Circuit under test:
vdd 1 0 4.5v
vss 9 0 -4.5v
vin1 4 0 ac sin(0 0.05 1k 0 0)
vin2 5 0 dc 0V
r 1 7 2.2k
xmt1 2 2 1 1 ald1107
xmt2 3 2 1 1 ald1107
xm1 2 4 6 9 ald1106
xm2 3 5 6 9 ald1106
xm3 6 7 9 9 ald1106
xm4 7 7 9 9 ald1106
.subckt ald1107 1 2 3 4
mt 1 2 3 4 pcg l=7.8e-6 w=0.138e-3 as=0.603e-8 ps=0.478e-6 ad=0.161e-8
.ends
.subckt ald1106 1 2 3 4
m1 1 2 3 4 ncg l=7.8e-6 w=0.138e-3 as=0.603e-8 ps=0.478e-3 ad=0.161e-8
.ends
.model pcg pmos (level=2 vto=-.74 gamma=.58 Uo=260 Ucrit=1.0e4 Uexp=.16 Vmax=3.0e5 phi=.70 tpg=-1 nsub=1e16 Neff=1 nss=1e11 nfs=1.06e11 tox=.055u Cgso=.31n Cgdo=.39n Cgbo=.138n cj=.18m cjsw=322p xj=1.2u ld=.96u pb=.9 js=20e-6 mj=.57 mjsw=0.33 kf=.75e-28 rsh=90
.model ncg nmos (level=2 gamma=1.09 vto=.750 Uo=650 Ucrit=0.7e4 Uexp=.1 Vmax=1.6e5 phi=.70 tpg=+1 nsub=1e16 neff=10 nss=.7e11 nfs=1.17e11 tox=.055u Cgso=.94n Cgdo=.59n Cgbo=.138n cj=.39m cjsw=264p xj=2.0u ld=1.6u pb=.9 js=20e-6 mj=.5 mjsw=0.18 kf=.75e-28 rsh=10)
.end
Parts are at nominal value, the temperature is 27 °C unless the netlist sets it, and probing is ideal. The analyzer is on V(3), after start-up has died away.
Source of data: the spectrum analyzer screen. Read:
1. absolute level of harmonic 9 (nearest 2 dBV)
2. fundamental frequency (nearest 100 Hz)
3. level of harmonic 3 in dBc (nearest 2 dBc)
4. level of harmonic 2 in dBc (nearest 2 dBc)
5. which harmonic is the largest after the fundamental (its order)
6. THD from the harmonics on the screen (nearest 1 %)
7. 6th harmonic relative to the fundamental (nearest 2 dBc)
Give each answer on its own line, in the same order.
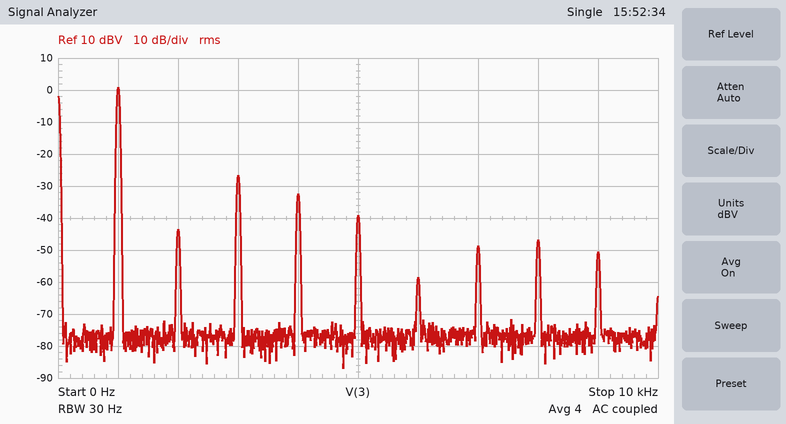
-50 dBV
1.0 kHz
-28 dBc
-44 dBc
3
5 %
-60 dBc
